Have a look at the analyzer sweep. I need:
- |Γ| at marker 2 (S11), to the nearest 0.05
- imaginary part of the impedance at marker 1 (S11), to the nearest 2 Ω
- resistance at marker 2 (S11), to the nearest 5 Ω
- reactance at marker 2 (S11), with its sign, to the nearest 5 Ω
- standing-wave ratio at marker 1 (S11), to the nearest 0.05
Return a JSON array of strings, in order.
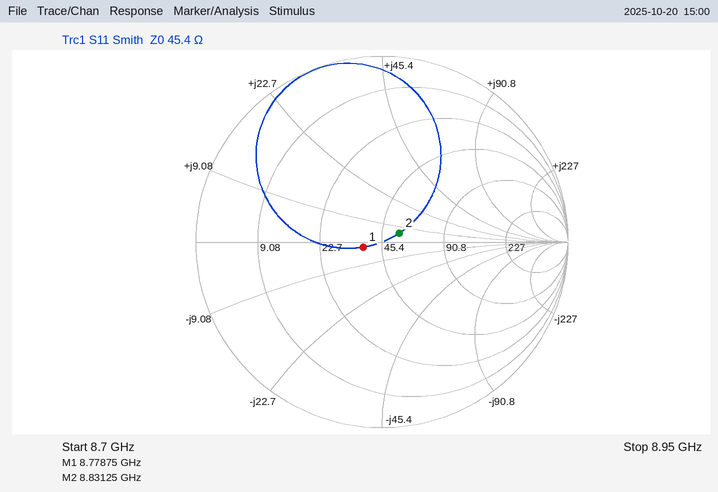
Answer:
["0.10", "-2 Ω", "55 Ω", "+5 Ω", "1.25"]
